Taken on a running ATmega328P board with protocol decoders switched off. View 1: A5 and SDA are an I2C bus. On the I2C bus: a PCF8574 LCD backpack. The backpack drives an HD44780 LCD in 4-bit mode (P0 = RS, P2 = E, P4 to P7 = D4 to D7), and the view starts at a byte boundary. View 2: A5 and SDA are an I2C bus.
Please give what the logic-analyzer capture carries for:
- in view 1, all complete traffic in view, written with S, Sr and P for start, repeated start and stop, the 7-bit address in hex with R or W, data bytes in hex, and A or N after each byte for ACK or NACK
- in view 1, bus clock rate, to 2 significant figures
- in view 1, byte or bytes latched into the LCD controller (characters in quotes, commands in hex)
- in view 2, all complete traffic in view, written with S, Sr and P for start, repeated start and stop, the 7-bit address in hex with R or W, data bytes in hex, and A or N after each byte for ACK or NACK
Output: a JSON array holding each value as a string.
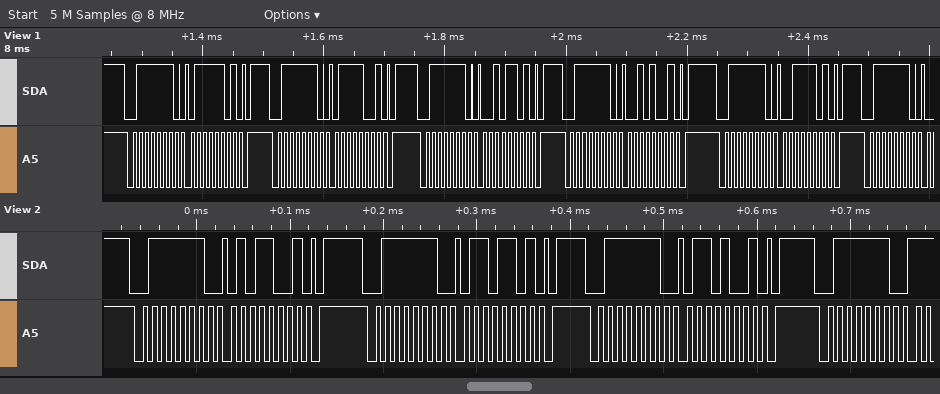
["S 3FW A 7D A P S 3FW A 79 A P S 3FW A 2D A P S 3FW A 29 A P S 3FW A 3D A P S 3FW A", "100 kHz", "'r'", "S 3FW A 59 A P S 3FW A 6D A P S 3FW A 69 A P S 3FW A"]
